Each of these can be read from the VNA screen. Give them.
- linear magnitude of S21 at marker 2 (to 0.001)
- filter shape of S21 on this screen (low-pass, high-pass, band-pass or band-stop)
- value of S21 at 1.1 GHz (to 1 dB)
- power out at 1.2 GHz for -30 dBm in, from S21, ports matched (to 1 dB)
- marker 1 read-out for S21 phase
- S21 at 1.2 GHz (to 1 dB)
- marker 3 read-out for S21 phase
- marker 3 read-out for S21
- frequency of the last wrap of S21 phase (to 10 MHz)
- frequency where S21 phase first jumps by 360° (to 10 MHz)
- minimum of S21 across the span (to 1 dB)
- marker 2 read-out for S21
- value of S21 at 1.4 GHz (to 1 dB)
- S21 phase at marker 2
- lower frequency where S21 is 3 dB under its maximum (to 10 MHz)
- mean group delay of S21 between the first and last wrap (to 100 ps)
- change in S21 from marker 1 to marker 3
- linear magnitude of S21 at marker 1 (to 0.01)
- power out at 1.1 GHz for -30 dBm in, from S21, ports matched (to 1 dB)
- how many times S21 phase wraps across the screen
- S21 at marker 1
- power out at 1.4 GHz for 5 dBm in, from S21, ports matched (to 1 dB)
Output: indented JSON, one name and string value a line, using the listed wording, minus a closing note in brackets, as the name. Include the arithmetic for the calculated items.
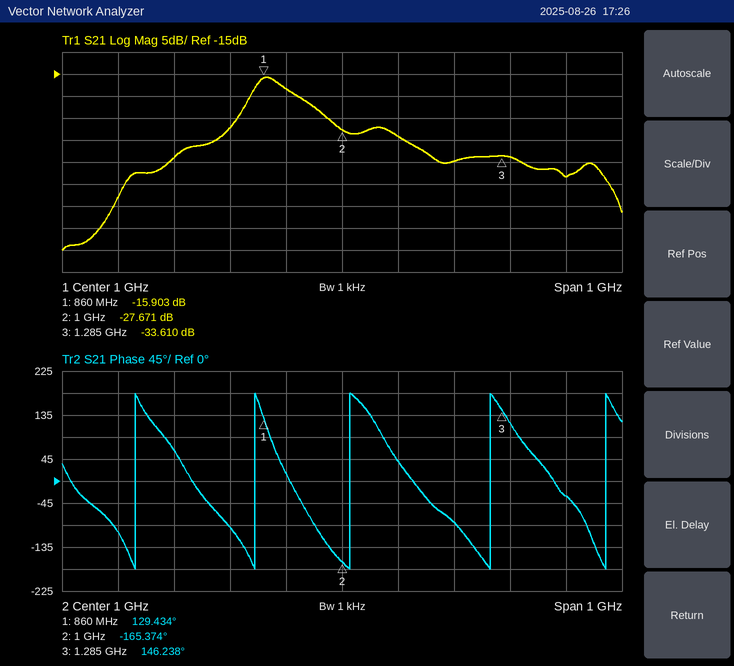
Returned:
{
  "linear magnitude of S21 at marker 2": "10^(-27.671/20) ≈ 0.041",
  "filter shape of S21 on this screen": "band-pass",
  "value of S21 at 1.1 GHz": "-29 dB",
  "power out at 1.2 GHz for -30 dBm in, from S21, ports matched": "-30 dBm + (-35 dB) = -65 dBm",
  "marker 1 read-out for S21 phase": "129.434°",
  "S21 at 1.2 GHz": "-35 dB",
  "marker 3 read-out for S21 phase": "146.238°",
  "marker 3 read-out for S21": "-33.610 dB",
  "frequency of the last wrap of S21 phase": "1.47 GHz",
  "frequency where S21 phase first jumps by 360°": "630 MHz",
  "minimum of S21 across the span": "-55 dB",
  "marker 2 read-out for S21": "-27.671 dB",
  "value of S21 at 1.4 GHz": "-38 dB",
  "S21 phase at marker 2": "-165.374°",
  "lower frequency where S21 is 3 dB under its maximum": "840 MHz",
  "mean group delay of S21 between the first and last wrap": "4 cycles / (1.47 GHz − 630 MHz) ≈ 4.8 ns",
  "change in S21 from marker 1 to marker 3": "-33.61 − (-15.903) = -17.707 dB",
  "linear magnitude of S21 at marker 1": "10^(-15.903/20) ≈ 0.16",
  "power out at 1.1 GHz for -30 dBm in, from S21, ports matched": "-30 dBm + (-29 dB) = -59 dBm",
  "how many times S21 phase wraps across the screen": "5",
  "S21 at marker 1": "-15.903 dB",
  "power out at 1.4 GHz for 5 dBm in, from S21, ports matched": "5 dBm + (-38 dB) = -33 dBm"
}
